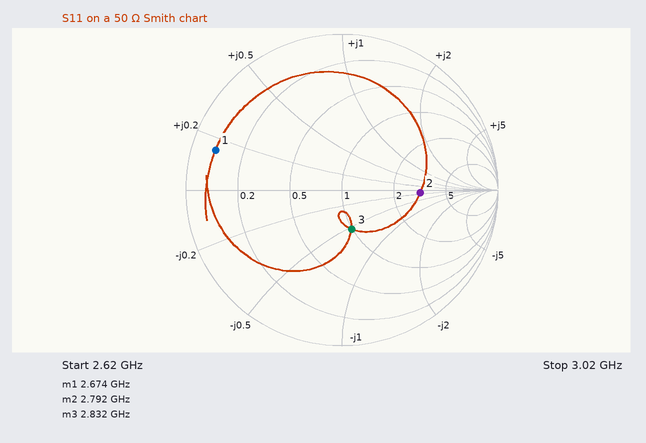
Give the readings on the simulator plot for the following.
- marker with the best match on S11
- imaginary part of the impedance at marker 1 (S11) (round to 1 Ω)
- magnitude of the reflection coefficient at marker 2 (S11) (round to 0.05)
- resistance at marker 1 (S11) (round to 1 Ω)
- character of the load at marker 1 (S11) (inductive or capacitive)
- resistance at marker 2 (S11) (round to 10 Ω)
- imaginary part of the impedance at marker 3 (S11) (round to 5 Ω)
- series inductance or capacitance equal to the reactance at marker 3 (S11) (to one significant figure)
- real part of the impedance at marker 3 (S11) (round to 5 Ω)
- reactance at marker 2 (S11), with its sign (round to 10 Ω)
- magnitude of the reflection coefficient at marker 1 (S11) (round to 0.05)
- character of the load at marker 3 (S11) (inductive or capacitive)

marker 3
+8 Ω
0.50
4 Ω
inductive
150 Ω
-25 Ω
2 pF
50 Ω
-10 Ω
0.85
capacitive
